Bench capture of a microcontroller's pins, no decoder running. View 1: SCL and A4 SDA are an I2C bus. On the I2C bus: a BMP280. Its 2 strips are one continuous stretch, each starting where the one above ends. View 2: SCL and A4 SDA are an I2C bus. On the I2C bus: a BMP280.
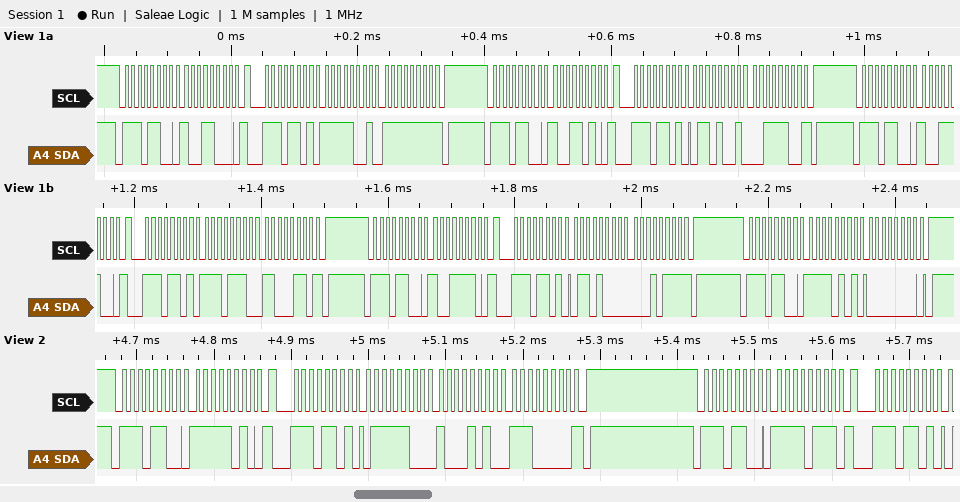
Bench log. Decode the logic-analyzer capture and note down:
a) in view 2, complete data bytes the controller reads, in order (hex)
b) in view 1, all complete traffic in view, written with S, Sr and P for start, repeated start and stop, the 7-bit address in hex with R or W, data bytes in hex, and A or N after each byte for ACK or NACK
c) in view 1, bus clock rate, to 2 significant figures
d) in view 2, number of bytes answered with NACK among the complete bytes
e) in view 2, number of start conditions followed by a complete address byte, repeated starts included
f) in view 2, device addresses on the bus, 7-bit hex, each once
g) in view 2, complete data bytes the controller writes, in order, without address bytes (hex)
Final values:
7C 8A E0
S 76W A 98 A Sr 76R A F9 A FF N P S 76W A 9A A Sr 76R A 69 A 3C N P S 76W A 9C A Sr 76R A EE A C6 N P S 76W A 9E A Sr 76R A 68 A 17 N P S 76W A F5 A 00 A P
100 kHz
1
4
0x76
FA F7
